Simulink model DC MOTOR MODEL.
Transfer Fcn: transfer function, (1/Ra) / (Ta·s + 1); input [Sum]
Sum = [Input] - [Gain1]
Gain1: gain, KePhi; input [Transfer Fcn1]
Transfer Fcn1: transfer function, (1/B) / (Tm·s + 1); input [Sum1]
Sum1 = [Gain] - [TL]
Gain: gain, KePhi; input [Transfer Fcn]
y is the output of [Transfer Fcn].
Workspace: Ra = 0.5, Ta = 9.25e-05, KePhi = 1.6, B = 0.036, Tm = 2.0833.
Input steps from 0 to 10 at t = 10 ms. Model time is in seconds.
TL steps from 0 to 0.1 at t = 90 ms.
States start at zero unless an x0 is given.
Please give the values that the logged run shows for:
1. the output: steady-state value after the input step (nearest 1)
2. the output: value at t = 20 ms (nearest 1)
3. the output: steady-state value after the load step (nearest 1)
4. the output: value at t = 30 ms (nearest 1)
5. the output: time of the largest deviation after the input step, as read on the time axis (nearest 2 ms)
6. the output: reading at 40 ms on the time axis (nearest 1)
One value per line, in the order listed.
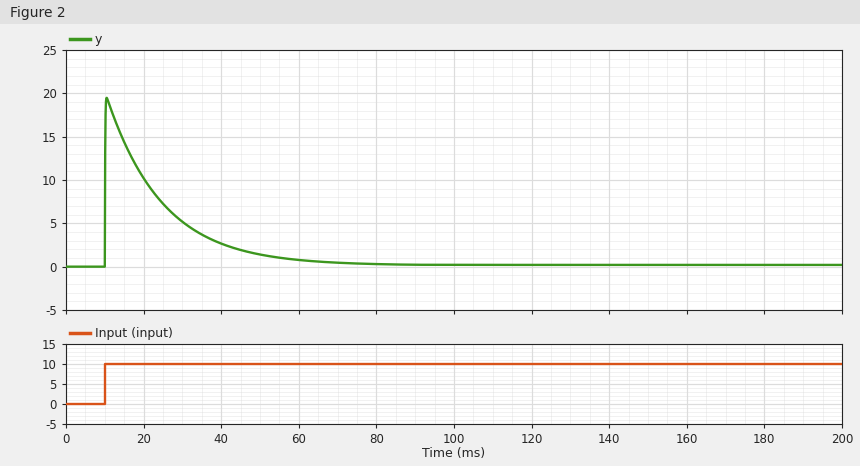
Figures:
0
10
0
5
10 ms
3
